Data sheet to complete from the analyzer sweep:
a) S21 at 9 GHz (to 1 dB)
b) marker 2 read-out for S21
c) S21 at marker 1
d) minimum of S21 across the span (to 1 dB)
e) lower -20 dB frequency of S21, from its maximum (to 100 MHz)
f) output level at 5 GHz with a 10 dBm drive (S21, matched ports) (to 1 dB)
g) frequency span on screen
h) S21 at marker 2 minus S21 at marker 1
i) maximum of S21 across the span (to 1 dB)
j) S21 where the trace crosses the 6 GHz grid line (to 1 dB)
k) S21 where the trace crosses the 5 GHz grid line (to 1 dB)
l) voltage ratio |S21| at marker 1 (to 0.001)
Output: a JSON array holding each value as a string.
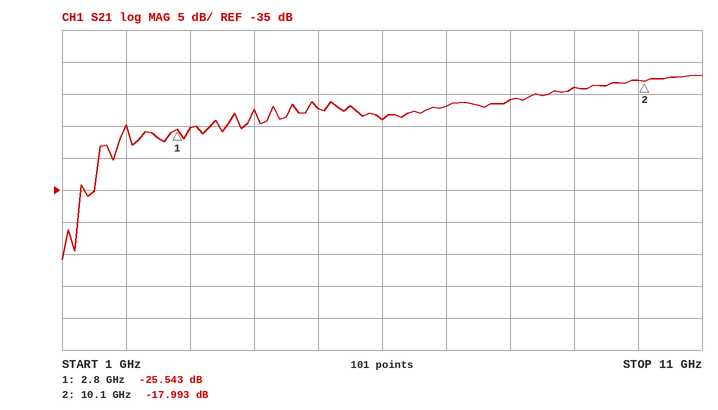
["-19 dB", "-17.993 dB", "-25.543 dB", "-46 dB", "1.3 GHz", "-12 dBm", "10 GHz", "7.550 dB", "-17 dB", "-24 dB", "-22 dB", "0.053"]
